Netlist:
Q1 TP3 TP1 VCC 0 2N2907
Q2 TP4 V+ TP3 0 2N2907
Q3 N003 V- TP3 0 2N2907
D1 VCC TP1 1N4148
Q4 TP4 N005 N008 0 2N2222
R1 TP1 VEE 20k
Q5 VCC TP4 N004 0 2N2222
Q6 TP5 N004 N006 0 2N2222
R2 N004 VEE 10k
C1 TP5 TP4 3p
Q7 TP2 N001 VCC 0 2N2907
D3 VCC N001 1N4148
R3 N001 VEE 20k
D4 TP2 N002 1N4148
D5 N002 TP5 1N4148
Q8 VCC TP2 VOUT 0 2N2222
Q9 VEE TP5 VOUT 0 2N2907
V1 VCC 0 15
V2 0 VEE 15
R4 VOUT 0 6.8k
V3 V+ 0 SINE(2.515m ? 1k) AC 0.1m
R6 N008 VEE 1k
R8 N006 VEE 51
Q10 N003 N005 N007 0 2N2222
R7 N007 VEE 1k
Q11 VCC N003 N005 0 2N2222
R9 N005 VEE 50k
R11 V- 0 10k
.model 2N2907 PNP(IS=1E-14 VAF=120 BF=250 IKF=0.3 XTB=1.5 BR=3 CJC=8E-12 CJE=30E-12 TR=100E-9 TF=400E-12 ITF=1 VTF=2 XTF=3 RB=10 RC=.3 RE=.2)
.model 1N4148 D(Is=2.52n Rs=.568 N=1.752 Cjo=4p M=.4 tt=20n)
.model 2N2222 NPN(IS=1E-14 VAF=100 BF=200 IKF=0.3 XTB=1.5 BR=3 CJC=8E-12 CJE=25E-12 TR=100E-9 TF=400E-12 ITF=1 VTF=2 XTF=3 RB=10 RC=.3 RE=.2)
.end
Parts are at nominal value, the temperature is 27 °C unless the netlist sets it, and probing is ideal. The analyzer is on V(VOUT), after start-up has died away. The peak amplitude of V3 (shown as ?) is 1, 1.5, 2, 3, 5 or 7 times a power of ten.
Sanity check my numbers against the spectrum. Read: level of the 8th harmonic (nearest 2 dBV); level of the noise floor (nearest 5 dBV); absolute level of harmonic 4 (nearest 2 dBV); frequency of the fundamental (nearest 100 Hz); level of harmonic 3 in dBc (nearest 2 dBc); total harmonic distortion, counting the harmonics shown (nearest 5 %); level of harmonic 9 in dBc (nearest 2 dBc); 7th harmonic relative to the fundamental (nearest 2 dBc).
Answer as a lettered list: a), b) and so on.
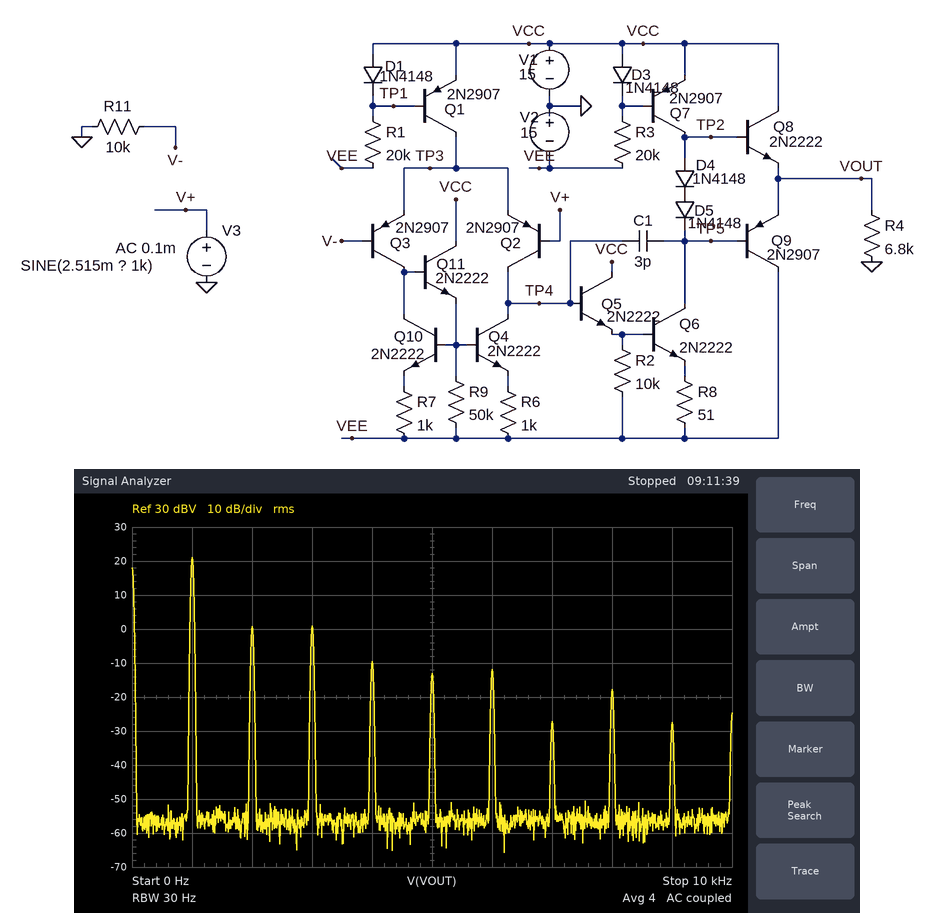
a) -18 dBV
b) -55 dBV
c) -10 dBV
d) 1.0 kHz
e) -20 dBc
f) 15 %
g) -48 dBc
h) -48 dBc
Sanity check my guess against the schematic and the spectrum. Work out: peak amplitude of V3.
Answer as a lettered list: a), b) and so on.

a) 150 µV
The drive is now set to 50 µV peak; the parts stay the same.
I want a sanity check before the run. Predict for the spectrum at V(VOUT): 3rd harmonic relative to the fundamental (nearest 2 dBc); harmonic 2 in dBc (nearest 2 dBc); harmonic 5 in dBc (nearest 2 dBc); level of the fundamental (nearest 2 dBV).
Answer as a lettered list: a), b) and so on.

a) -22 dBc
b) -12 dBc
c) -32 dBc
d) 10 dBV
